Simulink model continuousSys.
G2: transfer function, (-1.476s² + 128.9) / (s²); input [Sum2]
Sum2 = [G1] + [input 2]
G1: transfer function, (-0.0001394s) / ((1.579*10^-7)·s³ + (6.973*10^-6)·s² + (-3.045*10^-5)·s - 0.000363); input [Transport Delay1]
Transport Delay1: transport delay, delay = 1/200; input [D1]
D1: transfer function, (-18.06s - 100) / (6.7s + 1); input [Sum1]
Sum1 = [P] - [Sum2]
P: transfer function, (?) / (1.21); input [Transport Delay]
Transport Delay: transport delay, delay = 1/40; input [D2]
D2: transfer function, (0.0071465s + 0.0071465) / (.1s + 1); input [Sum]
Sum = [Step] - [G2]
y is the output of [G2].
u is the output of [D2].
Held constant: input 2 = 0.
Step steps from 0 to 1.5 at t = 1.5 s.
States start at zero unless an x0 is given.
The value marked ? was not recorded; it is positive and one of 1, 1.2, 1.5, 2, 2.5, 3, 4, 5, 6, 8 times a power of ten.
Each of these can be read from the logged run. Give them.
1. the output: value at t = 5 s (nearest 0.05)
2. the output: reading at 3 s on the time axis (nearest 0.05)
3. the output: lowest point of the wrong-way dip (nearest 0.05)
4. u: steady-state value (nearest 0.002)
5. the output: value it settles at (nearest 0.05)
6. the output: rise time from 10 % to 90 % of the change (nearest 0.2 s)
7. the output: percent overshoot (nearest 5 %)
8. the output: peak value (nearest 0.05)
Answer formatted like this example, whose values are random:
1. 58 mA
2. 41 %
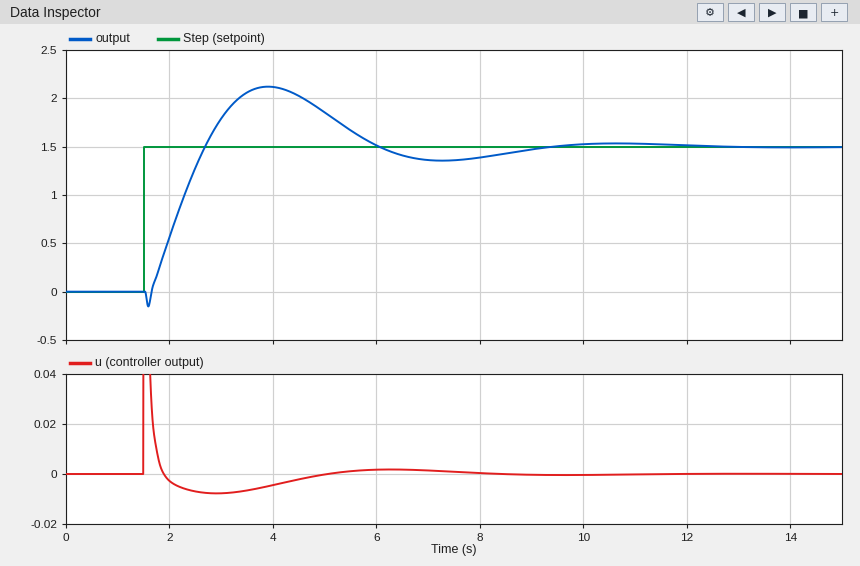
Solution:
1. 1.85
2. 1.80
3. -0.15
4. 0.000
5. 1.50
6. 0.8 s
7. 40 %
8. 2.10
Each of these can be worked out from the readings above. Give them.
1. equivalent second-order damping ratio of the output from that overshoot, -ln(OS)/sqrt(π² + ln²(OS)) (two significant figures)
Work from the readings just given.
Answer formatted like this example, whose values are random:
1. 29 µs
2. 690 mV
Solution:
1. 0.28
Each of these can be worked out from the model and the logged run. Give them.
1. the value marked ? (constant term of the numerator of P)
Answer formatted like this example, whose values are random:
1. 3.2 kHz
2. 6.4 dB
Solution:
1. 1
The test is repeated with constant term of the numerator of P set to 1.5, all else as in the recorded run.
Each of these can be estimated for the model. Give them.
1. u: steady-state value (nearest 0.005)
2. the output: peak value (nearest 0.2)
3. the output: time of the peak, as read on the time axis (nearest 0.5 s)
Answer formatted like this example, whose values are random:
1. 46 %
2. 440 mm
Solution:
1. 0.000
2. 2.0
3. 3.5 s
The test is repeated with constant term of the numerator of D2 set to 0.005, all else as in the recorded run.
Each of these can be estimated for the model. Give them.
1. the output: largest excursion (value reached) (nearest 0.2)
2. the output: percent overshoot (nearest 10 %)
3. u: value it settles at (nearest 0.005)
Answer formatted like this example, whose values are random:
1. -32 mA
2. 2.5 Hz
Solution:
1. 2.0
2. 30 %
3. 0.000
